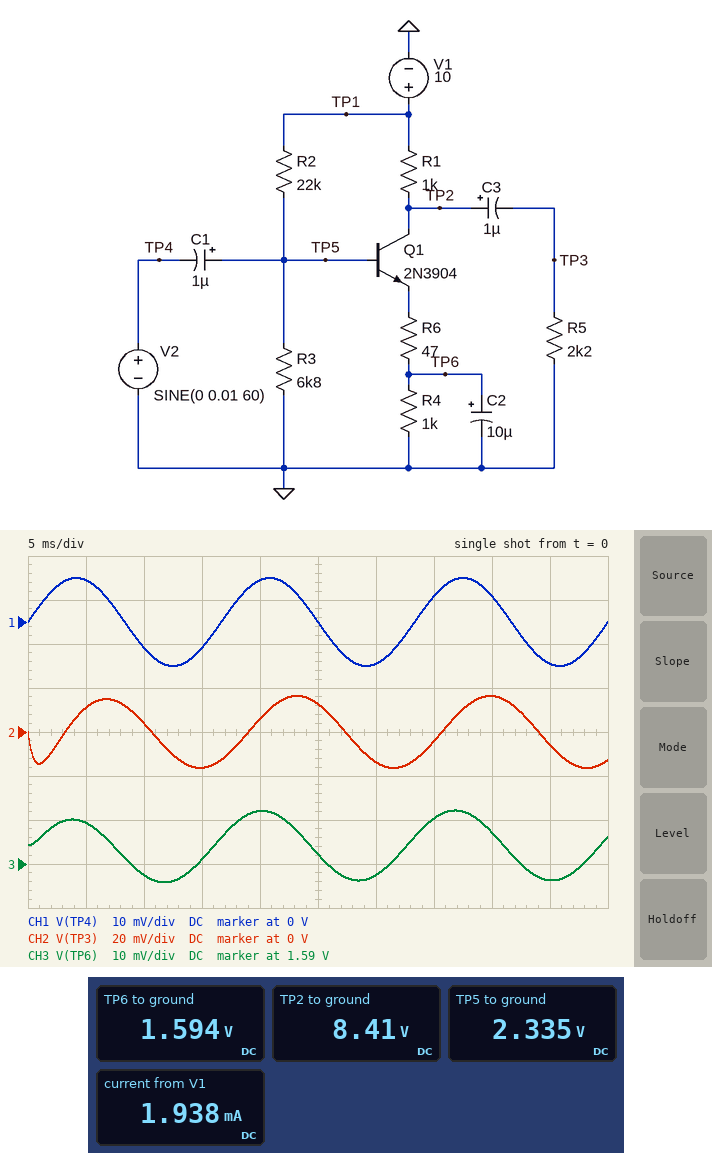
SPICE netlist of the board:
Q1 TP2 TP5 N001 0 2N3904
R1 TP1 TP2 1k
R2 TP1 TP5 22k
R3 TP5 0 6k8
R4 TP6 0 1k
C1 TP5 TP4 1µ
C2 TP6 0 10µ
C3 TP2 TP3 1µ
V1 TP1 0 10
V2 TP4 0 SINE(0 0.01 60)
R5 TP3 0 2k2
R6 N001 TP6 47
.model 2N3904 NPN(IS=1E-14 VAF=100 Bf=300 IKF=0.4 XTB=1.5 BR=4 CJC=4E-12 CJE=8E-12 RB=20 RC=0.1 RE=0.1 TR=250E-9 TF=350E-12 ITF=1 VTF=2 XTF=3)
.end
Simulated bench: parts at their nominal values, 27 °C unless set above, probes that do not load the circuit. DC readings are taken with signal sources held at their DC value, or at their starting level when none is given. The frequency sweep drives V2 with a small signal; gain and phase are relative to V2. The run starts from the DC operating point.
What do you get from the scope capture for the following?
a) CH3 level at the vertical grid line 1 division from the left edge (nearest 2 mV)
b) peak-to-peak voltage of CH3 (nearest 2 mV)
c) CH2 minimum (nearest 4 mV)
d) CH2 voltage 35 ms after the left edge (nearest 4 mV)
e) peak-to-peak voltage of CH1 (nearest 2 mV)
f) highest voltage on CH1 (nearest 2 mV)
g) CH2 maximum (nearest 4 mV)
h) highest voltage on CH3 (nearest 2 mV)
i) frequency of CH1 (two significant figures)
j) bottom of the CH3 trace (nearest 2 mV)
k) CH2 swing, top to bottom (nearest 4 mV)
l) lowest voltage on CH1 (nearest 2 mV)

1.600 V
16 mV
-16 mV
-4 mV
20 mV
10 mV
16 mV
1.602 V
60 Hz
1.586 V
32 mV
-10 mV
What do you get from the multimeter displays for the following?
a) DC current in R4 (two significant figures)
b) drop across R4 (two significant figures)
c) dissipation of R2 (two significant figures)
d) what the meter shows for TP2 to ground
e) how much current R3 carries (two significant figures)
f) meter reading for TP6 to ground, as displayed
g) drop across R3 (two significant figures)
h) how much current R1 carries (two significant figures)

1.6 mA
1.6 V
2.7 mW
8.41 V
340 µA
1.594 V
2.3 V
1.6 mA
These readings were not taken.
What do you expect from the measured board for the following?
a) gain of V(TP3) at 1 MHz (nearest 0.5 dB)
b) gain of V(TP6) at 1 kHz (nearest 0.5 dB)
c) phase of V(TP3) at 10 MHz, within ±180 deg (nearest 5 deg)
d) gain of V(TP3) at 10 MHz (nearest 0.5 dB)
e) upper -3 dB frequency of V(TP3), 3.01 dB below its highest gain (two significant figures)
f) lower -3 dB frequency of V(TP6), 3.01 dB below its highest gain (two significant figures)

20.5 dB
-12.5 dB
170 deg
20.5 dB
80 MHz
25 Hz
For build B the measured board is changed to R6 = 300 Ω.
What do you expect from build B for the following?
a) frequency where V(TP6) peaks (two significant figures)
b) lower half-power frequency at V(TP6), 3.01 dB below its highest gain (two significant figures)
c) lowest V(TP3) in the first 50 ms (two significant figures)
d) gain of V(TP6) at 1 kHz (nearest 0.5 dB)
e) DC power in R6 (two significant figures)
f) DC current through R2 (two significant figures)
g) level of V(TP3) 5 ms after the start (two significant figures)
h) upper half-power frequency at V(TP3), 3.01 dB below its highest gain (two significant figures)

45 Hz
18 Hz
-10 mV
-26.0 dB
500 µW
350 µA
2.7 mV
170 MHz
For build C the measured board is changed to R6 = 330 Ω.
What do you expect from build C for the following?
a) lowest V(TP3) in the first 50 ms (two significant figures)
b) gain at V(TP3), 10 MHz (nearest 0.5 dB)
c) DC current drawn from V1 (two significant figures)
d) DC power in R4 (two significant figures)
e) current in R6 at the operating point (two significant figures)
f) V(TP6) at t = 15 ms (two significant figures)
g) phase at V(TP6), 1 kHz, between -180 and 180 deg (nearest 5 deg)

-9.6 mV
6.0 dB
1.6 mA
1.6 mW
1.3 mA
1.3 V
-85 deg
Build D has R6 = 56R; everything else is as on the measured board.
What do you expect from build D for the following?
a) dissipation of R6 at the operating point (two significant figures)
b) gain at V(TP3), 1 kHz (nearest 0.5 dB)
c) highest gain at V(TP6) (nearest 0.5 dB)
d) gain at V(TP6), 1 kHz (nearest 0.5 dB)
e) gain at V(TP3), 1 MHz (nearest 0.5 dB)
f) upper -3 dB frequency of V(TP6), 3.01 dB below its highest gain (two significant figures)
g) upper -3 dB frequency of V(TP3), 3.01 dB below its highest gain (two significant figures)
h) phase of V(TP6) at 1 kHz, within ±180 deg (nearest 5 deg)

140 µW
19.0 dB
-2.0 dB
-13.5 dB
19.5 dB
300 Hz
83 MHz
-75 deg
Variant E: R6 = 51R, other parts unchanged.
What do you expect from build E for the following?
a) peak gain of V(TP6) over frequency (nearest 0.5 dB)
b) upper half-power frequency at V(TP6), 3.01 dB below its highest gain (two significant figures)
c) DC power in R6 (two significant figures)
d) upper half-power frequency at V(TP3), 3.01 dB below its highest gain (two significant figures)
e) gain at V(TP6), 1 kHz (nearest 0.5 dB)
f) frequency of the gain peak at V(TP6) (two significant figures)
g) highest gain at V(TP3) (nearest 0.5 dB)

-2.0 dB
310 Hz
130 µW
82 MHz
-13.0 dB
88 Hz
20.0 dB
